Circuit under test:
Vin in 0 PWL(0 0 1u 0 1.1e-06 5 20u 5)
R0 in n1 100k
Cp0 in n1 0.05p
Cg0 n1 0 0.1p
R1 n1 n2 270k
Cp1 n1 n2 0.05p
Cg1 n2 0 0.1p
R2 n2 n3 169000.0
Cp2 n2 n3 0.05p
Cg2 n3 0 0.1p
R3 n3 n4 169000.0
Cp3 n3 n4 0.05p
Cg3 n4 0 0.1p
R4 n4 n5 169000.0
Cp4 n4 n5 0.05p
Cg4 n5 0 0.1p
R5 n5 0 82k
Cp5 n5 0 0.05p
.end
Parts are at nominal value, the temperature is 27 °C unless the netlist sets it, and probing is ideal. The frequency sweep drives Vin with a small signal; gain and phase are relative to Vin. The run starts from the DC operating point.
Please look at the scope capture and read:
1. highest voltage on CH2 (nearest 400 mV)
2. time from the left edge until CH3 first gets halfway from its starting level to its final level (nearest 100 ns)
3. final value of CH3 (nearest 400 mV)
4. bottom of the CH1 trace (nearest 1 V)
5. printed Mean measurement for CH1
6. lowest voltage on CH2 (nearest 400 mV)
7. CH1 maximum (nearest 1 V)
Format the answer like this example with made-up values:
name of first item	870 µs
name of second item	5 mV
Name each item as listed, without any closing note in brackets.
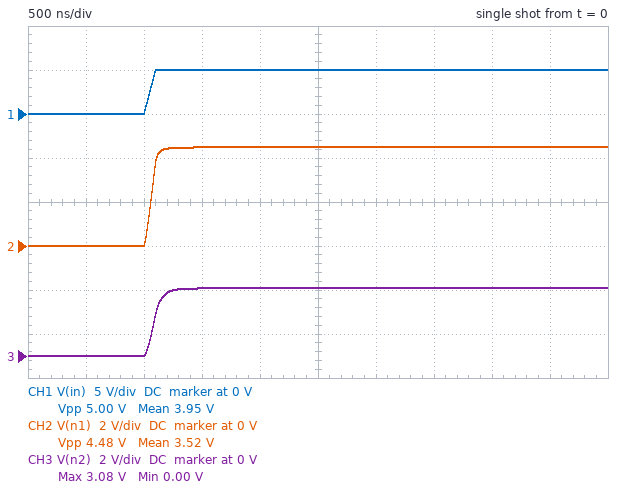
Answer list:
highest voltage on CH2	4.4 V
time from the left edge until CH3 first gets halfway from its starting level to its final level	1.1 µs
final value of CH3	3.2 V
bottom of the CH1 trace	0 V
printed Mean measurement for CH1	3.95 V
lowest voltage on CH2	0 V
CH1 maximum	5 V
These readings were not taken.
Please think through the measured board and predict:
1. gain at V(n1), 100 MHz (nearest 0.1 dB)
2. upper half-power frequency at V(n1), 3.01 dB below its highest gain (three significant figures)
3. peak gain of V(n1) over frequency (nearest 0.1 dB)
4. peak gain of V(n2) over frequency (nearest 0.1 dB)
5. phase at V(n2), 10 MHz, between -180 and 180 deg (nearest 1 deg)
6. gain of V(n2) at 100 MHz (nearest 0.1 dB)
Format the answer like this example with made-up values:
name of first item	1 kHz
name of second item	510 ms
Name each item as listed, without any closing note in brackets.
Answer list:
gain at V(n1), 100 MHz	-11.1 dB
upper half-power frequency at V(n1), 3.01 dB below its highest gain	9.20 MHz
peak gain of V(n1) over frequency	-1.0 dB
peak gain of V(n2) over frequency	-4.2 dB
phase at V(n2), 10 MHz, between -180 and 180 deg	-49 deg
gain of V(n2) at 100 MHz	-22.5 dB
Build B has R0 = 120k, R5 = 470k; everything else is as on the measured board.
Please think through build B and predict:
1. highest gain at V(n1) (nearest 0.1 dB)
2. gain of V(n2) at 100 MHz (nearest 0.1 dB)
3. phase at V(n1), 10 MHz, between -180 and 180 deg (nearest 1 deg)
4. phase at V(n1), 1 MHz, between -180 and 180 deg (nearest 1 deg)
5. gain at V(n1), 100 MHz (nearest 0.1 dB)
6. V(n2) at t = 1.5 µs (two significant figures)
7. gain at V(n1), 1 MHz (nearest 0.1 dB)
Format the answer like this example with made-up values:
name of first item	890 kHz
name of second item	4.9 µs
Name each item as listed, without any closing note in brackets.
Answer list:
highest gain at V(n1)	-0.8 dB
gain of V(n2) at 100 MHz	-22.6 dB
phase at V(n1), 10 MHz, between -180 and 180 deg	-28 deg
phase at V(n1), 1 MHz, between -180 and 180 deg	-8 deg
gain at V(n1), 100 MHz	-11.2 dB
V(n2) at t = 1.5 µs	3.5 V
gain at V(n1), 1 MHz	-1.2 dB
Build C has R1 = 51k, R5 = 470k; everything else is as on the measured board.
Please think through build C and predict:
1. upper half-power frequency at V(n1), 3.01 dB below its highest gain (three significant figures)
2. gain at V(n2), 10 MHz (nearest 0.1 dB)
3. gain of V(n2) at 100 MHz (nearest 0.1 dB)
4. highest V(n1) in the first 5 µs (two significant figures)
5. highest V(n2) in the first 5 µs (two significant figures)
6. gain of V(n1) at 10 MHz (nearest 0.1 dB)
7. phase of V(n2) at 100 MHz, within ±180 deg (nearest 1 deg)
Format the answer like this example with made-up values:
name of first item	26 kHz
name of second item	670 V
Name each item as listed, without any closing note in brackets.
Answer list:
upper half-power frequency at V(n1), 3.01 dB below its highest gain	5.05 MHz
gain at V(n2), 10 MHz	-8.4 dB
gain of V(n2) at 100 MHz	-21.4 dB
highest V(n1) in the first 5 µs	4.6 V
highest V(n2) in the first 5 µs	4.3 V
gain of V(n1) at 10 MHz	-6.1 dB
phase of V(n2) at 100 MHz, within ±180 deg	-29 deg
